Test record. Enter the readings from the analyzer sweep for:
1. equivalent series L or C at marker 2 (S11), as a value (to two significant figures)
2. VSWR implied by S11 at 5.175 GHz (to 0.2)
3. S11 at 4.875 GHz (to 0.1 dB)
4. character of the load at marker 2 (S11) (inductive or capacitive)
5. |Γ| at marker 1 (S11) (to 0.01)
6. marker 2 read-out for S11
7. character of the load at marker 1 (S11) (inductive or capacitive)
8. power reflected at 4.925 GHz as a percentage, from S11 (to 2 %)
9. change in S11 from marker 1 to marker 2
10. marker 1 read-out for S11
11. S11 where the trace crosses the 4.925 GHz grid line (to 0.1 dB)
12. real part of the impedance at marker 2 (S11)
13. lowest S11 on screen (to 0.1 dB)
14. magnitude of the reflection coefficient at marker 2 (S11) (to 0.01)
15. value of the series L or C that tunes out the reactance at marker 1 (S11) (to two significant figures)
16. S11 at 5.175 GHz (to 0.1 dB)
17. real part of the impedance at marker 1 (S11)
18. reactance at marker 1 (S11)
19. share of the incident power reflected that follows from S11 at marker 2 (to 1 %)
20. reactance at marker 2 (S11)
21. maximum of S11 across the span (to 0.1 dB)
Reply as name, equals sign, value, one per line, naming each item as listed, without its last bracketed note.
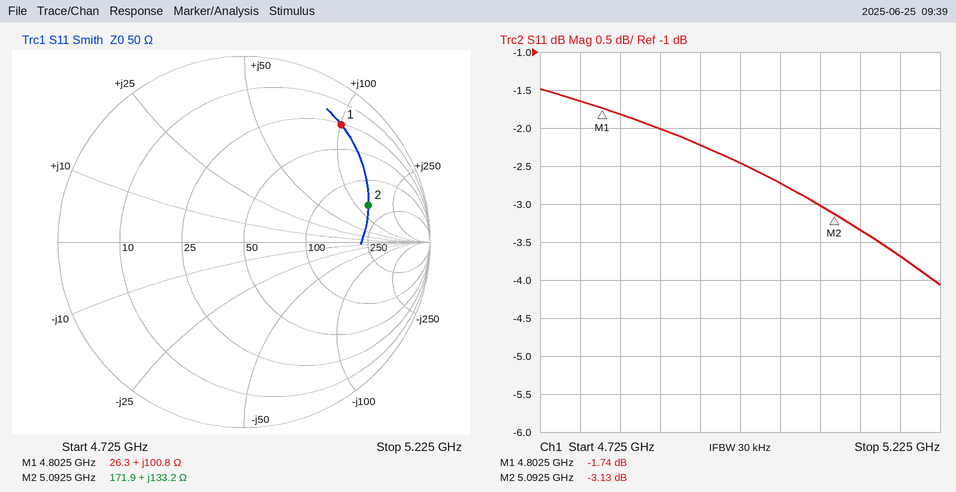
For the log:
equivalent series L or C at marker 2 (S11), as a value = 4.2 nH
VSWR implied by S11 at 5.175 GHz = 4.8
S11 at 4.875 GHz = -2.0 dB
character of the load at marker 2 (S11) = inductive
|Γ| at marker 1 (S11) = 0.82
marker 2 read-out for S11 = -3.13 dB
character of the load at marker 1 (S11) = inductive
power reflected at 4.925 GHz as a percentage, from S11 = 60 %
change in S11 from marker 1 to marker 2 = -1.39 dB
marker 1 read-out for S11 = -1.74 dB
S11 where the trace crosses the 4.925 GHz grid line = -2.2 dB
real part of the impedance at marker 2 = 171.9 Ω
lowest S11 on screen = -4.1 dB
magnitude of the reflection coefficient at marker 2 (S11) = 0.70
value of the series L or C that tunes out the reactance at marker 1 (S11) = 330 fF
S11 at 5.175 GHz = -3.7 dB
real part of the impedance at marker 1 = 26.3 Ω
reactance at marker 1 = +100.8 Ω
share of the incident power reflected that follows from S11 at marker 2 = 49 %
reactance at marker 2 = +133.2 Ω
maximum of S11 across the span = -1.5 dB
